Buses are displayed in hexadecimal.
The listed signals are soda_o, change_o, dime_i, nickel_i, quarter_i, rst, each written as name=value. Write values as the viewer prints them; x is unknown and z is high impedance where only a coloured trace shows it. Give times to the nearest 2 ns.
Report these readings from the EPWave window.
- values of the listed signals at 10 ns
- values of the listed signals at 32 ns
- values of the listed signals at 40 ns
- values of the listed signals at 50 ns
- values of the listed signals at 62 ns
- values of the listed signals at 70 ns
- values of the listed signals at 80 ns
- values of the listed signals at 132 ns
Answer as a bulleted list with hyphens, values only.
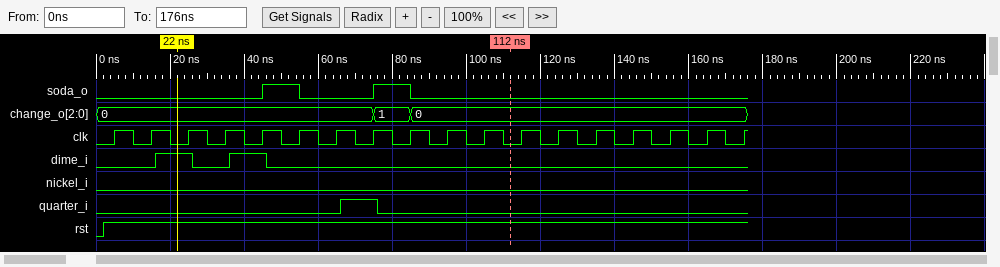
- soda_o=0, change_o=0, dime_i=0, nickel_i=0, quarter_i=0, rst=1
- soda_o=0, change_o=0, dime_i=0, nickel_i=0, quarter_i=0, rst=1
- soda_o=0, change_o=0, dime_i=1, nickel_i=0, quarter_i=0, rst=1
- soda_o=1, change_o=0, dime_i=0, nickel_i=0, quarter_i=0, rst=1
- soda_o=0, change_o=0, dime_i=0, nickel_i=0, quarter_i=0, rst=1
- soda_o=0, change_o=0, dime_i=0, nickel_i=0, quarter_i=1, rst=1
- soda_o=1, change_o=1, dime_i=0, nickel_i=0, quarter_i=0, rst=1
- soda_o=0, change_o=0, dime_i=0, nickel_i=0, quarter_i=0, rst=1
